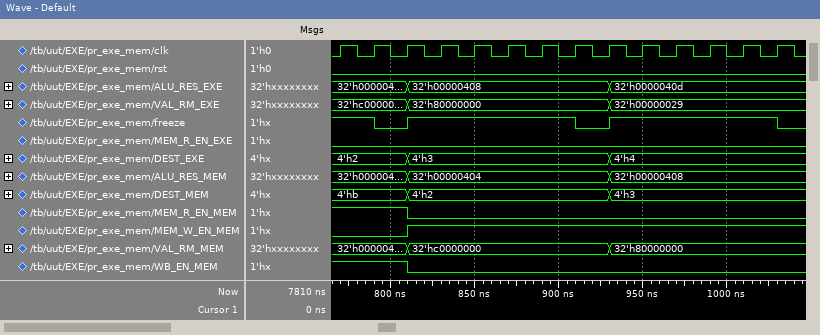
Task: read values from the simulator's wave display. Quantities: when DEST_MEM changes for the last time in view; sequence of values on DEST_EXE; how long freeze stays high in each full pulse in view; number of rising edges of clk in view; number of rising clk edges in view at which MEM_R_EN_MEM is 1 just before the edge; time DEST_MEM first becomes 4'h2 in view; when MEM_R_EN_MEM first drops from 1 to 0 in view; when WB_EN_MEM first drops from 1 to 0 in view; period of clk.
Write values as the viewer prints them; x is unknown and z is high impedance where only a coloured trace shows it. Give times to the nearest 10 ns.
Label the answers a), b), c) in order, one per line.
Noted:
a) 930 ns
b) 4'h2, 4'h3, 4'h4
c) 100 ns, 100 ns
d) 14
e) 3
f) 810 ns
g) 810 ns
h) 810 ns
i) 20 ns
